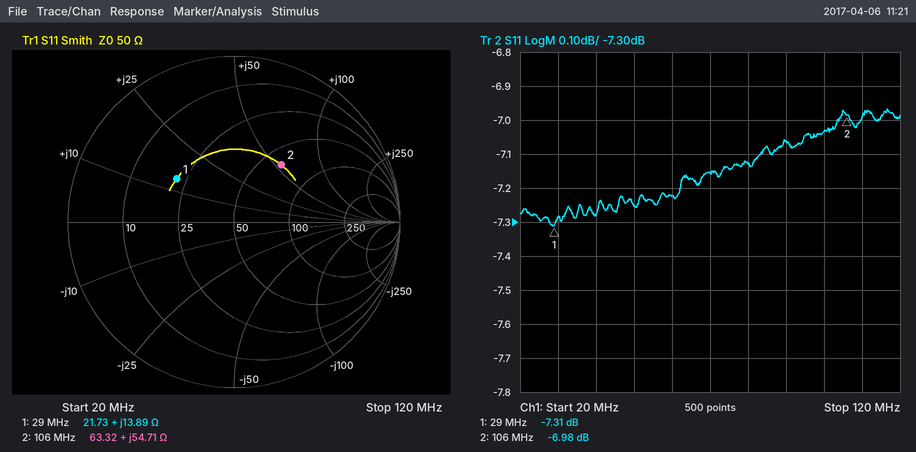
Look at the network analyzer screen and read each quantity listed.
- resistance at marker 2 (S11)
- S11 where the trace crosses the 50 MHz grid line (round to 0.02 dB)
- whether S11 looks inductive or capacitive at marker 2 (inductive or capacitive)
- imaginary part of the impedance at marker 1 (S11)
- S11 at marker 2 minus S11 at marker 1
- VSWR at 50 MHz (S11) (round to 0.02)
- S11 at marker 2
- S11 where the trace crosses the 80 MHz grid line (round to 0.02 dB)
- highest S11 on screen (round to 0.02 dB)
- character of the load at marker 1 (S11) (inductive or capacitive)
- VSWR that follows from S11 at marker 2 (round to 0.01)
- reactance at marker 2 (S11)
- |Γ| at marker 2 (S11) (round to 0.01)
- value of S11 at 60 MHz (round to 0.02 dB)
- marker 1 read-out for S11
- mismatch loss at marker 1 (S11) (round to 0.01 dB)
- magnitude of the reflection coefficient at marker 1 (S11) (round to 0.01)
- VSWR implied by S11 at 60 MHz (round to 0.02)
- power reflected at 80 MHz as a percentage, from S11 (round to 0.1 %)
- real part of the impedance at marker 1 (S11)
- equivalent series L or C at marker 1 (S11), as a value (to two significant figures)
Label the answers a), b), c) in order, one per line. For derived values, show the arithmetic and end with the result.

a) 63.32 Ω
b) -7.26 dB
c) inductive
d) +13.89 Ω
e) -6.98 − (-7.31) = 0.33 dB
f) |Γ| = 10^(-7.26/20) = 0.4335; VSWR = (1 + 0.4335)/(1 − 0.4335) ≈ 2.53, so 2.54 to the nearest 0.02
g) -6.98 dB
h) -7.12 dB
i) -6.96 dB
j) inductive
k) (1 + 0.4477)/(1 − 0.4477) ≈ 2.62
l) +54.71 Ω
m) 0.45
n) -7.22 dB
o) -7.31 dB
p) −10 log10(1 − 10^(-7.31/10)) ≈ 0.89 dB
q) 0.43
r) |Γ| = 10^(-7.22/20) = 0.4355; VSWR = (1 + 0.4355)/(1 − 0.4355) ≈ 2.54
s) 10^(-7.12/10) ≈ 19.4 %
t) 21.73 Ω
u) L = 13.89 Ω/(2π × 29 MHz) ≈ 76 nH
